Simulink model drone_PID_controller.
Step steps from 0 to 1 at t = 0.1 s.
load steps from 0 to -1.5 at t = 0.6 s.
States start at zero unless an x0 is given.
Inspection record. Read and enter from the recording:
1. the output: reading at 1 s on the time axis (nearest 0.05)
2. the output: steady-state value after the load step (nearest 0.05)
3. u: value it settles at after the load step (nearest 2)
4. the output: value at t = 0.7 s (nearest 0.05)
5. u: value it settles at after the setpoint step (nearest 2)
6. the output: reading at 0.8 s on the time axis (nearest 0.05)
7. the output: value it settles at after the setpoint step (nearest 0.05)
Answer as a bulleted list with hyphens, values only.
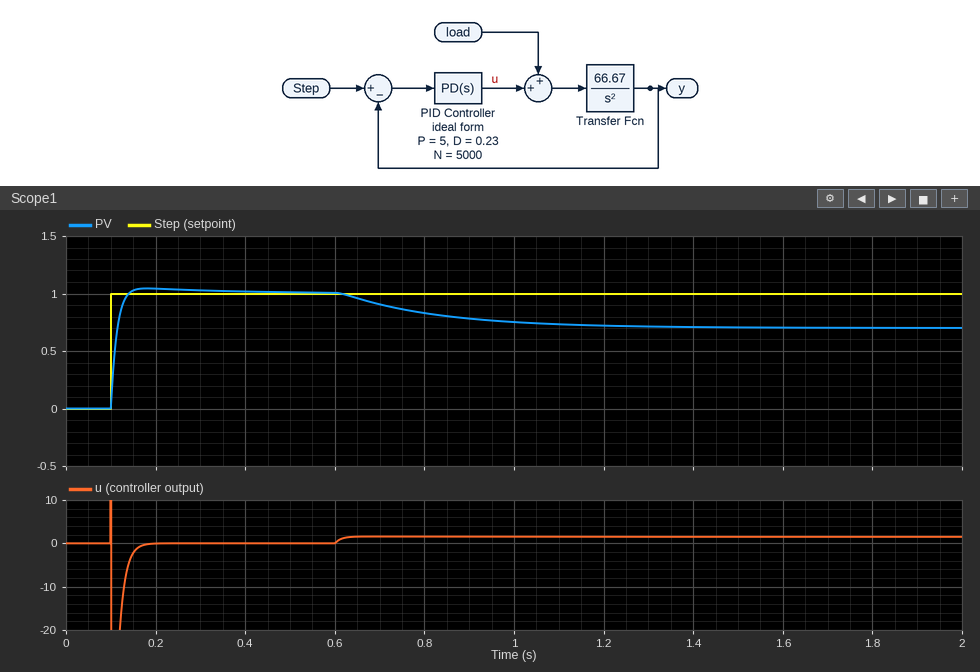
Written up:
- 0.75
- 0.70
- 2
- 0.90
- 0
- 0.85
- 1.00
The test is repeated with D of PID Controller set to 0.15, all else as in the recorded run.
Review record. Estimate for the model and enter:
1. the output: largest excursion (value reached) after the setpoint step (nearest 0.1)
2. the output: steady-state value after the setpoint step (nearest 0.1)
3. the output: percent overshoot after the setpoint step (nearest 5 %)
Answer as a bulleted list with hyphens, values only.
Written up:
- 1.1
- 1.0
- 10 %
